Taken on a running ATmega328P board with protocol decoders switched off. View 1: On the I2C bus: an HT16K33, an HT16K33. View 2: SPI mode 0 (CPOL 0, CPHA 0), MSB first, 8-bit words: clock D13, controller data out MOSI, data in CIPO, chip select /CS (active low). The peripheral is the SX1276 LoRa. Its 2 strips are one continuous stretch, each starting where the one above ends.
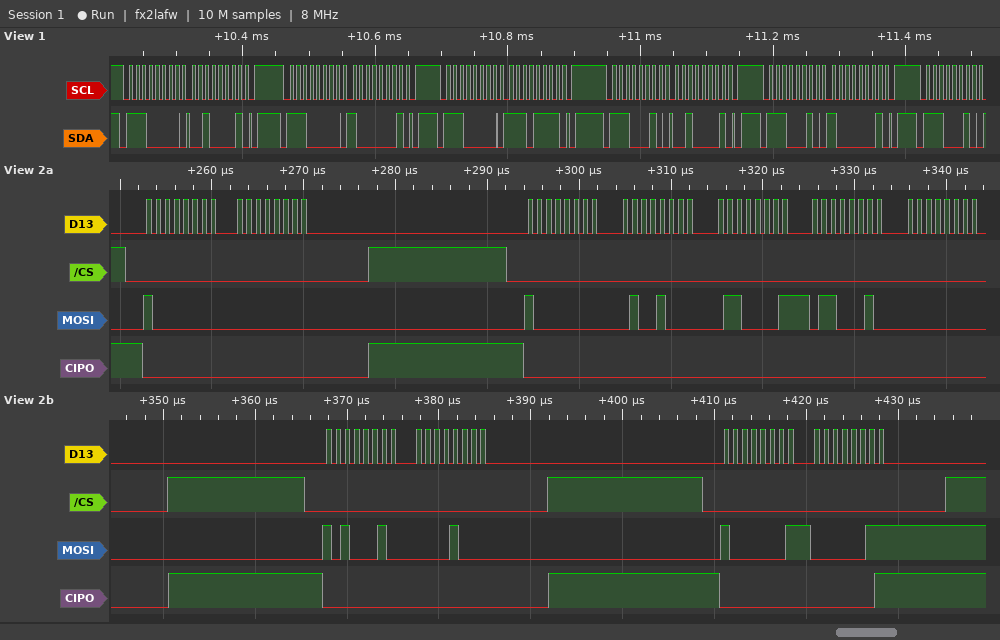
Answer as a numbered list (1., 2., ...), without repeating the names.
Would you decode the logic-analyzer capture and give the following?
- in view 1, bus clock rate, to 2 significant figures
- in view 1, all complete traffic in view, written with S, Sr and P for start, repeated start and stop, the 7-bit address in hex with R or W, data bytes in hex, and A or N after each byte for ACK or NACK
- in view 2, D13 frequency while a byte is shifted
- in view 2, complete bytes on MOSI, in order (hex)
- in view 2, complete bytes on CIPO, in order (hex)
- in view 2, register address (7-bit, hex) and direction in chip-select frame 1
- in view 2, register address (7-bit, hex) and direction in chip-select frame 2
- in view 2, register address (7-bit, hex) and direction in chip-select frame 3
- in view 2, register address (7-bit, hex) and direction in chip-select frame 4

1. 100 kHz
2. S 70W A 21 A P S 70W A 81 A P S 70W A EF A P S 71W A 21 A P S 71W A 81 A P S 71W A
3. 1 MHz
4. 80 00 80 48 61 62 00 A2 08 81 03
5. 00 00 00 00 00 00 00 00 00 00 01
6. 0x00 write
7. 0x00 write
8. 0x22 write
9. 0x01 write
